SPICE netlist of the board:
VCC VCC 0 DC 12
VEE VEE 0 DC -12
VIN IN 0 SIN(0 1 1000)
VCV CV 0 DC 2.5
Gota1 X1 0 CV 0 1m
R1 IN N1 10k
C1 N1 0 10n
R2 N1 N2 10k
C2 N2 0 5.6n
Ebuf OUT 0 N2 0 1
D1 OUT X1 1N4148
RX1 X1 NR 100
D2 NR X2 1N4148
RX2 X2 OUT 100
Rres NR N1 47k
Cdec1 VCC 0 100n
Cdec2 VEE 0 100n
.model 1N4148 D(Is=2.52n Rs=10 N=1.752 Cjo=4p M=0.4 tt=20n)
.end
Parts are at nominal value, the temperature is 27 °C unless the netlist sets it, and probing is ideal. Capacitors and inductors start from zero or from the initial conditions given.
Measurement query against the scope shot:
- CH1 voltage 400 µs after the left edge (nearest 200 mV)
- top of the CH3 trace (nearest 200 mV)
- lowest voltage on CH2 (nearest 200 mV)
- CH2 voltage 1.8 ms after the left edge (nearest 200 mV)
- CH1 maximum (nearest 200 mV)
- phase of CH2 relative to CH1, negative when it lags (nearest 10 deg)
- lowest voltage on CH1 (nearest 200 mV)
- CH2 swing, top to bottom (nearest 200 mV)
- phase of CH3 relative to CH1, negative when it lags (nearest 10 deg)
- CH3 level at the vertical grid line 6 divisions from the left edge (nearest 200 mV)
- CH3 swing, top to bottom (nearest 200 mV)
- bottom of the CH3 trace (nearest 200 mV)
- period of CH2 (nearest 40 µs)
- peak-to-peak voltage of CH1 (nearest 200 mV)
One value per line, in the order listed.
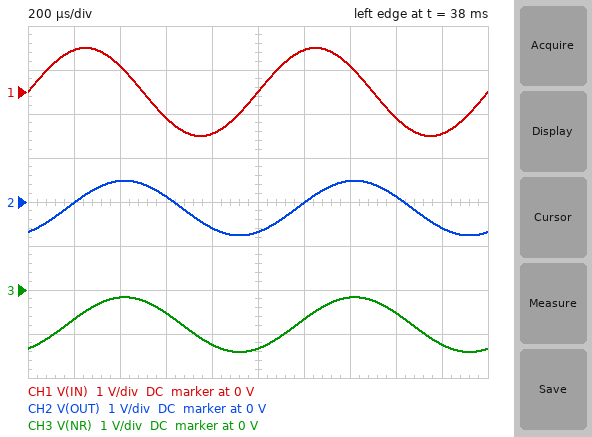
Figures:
600 mV
-200 mV
-800 mV
-600 mV
1.0 V
-60 deg
-1.0 V
1.2 V
-60 deg
-600 mV
1.2 V
-1.4 V
1.00 ms
2.0 V
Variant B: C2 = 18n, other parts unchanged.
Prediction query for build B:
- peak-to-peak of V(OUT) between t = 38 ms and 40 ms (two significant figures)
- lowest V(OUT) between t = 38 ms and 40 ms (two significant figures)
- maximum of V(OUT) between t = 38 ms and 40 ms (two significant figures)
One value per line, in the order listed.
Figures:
640 mV
-460 mV
180 mV
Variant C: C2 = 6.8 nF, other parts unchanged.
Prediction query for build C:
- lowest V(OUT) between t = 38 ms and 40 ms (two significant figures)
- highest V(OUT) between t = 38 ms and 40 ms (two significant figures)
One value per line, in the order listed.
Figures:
-710 mV
440 mV
